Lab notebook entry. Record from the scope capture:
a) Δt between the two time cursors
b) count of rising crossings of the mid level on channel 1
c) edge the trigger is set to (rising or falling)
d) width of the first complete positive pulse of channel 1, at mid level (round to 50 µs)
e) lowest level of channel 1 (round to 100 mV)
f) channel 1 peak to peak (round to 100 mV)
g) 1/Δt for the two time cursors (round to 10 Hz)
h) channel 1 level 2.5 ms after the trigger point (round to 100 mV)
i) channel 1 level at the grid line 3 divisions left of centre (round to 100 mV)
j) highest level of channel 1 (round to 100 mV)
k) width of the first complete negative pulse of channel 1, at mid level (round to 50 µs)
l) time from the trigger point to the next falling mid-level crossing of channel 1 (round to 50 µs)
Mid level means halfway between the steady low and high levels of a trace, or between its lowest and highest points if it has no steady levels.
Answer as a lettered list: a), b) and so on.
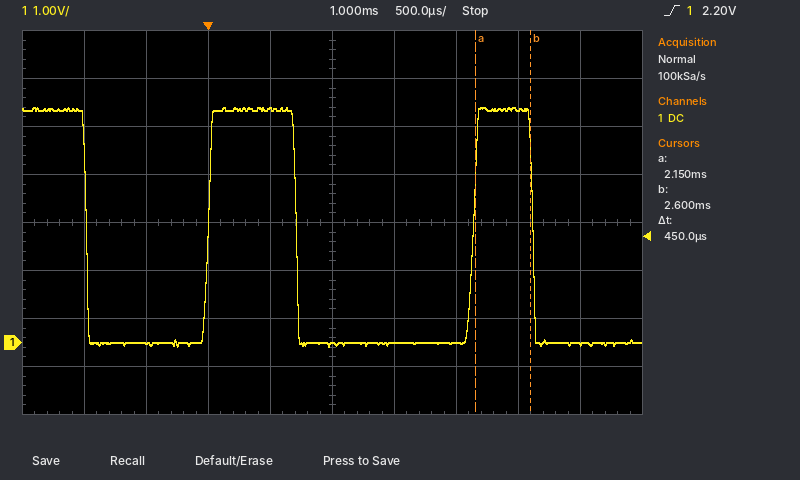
a) 450 µs
b) 2
c) rising
d) 700 µs
e) -100 mV
f) 5.0 V
g) 2.22 kHz
h) 4.9 V
i) 0.0 V
j) 4.9 V
k) 1.00 ms
l) 700 µs
